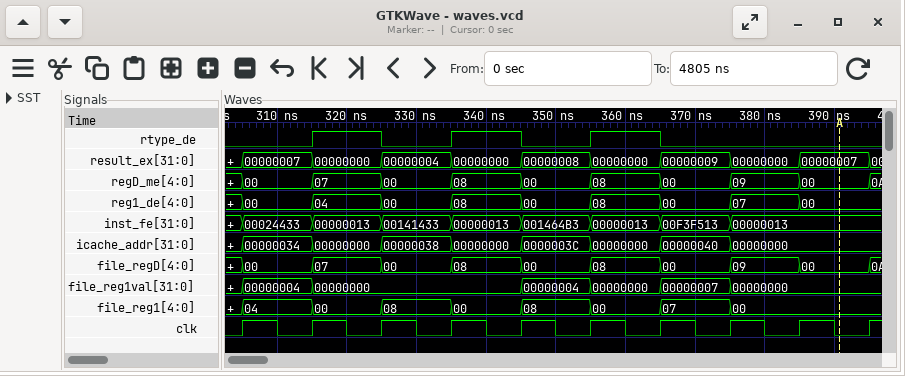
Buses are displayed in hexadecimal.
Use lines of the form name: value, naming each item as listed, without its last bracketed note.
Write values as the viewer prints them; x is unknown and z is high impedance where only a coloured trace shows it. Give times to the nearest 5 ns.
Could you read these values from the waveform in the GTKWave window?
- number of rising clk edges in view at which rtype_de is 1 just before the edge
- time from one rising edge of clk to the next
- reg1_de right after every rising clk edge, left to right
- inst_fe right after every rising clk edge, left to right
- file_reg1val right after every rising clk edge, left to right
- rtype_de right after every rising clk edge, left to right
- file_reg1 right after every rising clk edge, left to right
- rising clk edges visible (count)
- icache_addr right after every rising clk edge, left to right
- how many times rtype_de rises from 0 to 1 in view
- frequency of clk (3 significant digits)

number of rising clk edges in view at which rtype_de is 1 just before the edge: 3
time from one rising edge of clk to the next: 10 ns
reg1_de right after every rising clk edge, left to right: 00, 04, 00, 08, 00, 08, 00, 07, 00, 00
inst_fe right after every rising clk edge, left to right: 00024433, 00000013, 00141433, 00000013, 001464B3, 00000013, 00F3F513, 00000013, 00000013, 00000013
file_reg1val right after every rising clk edge, left to right: 00000004, 00000000, 00000000, 00000000, 00000004, 00000000, 00000007, 00000000, 00000000, 00000000
rtype_de right after every rising clk edge, left to right: 0 1 0 1 0 1 0 0 0 0
file_reg1 right after every rising clk edge, left to right: 04, 00, 08, 00, 08, 00, 07, 00, 00, 00
rising clk edges visible: 10
icache_addr right after every rising clk edge, left to right: 00000034, 00000000, 00000038, 00000000, 0000003C, 00000000, 00000040, 00000000, 00000000, 00000000
how many times rtype_de rises from 0 to 1 in view: 3
frequency of clk: 100 MHz
